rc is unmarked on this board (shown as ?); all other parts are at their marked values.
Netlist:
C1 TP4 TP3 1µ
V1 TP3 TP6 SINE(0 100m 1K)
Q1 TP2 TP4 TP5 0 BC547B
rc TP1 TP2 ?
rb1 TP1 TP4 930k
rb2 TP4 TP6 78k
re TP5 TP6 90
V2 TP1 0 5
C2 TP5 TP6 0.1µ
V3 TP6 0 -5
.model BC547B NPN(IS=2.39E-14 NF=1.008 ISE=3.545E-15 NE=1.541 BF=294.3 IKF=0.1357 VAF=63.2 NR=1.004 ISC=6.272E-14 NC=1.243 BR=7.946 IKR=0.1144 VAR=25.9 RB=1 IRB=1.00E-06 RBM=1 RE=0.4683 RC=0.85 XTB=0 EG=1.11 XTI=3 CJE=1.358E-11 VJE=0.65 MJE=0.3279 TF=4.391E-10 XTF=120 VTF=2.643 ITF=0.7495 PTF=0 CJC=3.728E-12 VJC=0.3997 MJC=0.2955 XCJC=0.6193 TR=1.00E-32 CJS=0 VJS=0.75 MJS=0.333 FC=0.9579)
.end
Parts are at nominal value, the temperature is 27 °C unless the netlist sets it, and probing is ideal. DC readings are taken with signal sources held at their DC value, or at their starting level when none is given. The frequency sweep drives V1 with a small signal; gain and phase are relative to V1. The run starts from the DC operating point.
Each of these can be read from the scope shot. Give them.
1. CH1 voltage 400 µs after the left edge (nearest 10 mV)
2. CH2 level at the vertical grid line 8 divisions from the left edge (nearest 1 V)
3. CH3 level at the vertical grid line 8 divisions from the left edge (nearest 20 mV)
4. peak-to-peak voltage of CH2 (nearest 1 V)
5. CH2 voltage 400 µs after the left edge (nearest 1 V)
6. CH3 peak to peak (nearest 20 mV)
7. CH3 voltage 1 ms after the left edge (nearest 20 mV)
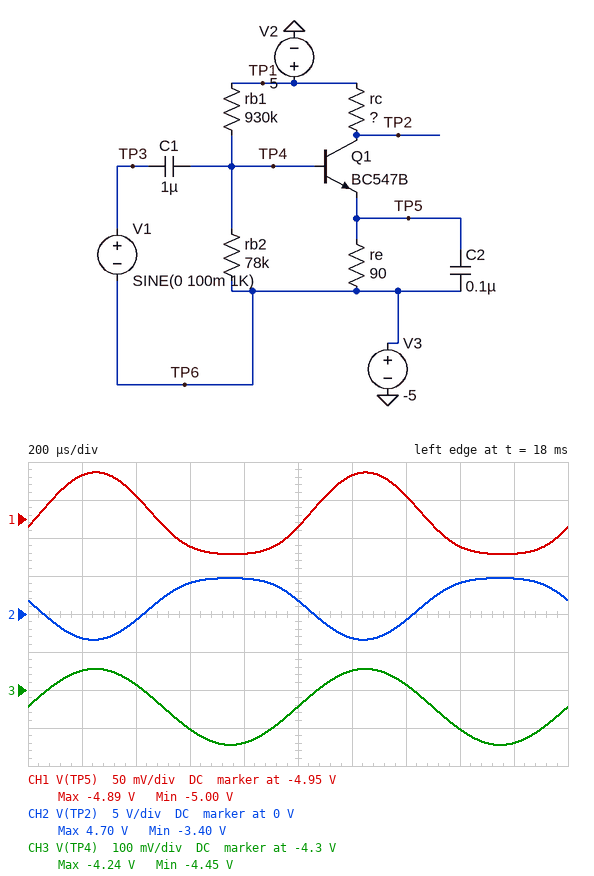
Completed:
-4.92 V
4 V
-4.40 V
8 V
-1 V
200 mV
-4.34 V
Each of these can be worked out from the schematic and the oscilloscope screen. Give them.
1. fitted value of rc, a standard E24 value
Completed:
6.8 kΩ
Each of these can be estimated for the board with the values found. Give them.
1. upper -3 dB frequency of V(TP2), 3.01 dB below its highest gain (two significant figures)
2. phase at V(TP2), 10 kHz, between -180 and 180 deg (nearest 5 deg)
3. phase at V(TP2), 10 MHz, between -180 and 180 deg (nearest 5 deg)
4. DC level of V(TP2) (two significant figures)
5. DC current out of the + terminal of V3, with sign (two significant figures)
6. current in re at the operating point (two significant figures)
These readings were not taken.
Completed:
15 MHz
-165 deg
145 deg
1.7 V
-500 µA
490 µA
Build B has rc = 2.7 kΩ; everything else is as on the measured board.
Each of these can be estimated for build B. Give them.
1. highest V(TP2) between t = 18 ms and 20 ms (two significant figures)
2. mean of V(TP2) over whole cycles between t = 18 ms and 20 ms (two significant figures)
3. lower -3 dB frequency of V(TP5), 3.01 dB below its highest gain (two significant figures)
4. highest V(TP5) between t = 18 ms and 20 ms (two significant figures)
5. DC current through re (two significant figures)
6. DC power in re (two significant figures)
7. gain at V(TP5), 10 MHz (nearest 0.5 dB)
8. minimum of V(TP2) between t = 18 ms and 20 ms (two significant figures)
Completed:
4.9 V
3.5 V
5.7 Hz
-4.9 V
500 µA
22 µW
-50.5 dB
1.6 V
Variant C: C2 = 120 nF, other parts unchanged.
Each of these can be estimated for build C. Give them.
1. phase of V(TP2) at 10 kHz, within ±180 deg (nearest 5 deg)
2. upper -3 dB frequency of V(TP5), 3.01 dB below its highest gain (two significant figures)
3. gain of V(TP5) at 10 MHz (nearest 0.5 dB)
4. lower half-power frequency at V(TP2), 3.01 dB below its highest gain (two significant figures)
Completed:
-160 deg
38 kHz
-52.5 dB
32 kHz
